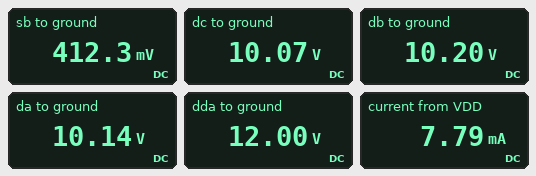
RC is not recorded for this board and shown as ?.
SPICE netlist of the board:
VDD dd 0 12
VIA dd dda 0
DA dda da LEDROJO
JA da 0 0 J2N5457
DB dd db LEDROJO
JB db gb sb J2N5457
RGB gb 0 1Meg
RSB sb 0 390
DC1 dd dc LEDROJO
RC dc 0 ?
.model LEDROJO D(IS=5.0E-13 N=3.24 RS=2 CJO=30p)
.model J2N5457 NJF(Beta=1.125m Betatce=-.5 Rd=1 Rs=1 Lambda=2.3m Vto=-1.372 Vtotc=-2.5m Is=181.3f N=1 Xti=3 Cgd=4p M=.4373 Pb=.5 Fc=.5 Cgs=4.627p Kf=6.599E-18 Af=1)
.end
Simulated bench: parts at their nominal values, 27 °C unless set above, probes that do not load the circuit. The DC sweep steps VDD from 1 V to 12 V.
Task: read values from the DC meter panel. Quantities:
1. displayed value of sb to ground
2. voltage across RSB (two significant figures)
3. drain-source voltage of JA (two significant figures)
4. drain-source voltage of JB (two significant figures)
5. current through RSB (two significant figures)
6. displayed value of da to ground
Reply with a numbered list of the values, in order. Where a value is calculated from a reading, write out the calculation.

1. 412.3 mV
2. 412.3 mV = 410 mV
3. 10.14 V = 10 V
4. 10.2 V - 412.3 mV = 9.8 V
5. (412.3 mV) / 390 Ω = 1.1 mA
6. 10.14 V
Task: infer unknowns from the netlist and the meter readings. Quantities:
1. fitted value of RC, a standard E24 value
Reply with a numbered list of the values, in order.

1. 2.2 kΩ
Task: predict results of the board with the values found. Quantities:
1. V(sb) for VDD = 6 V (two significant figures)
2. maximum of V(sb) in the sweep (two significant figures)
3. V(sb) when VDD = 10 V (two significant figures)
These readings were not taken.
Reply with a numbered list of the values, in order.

1. 410 mV
2. 410 mV
3. 410 mV
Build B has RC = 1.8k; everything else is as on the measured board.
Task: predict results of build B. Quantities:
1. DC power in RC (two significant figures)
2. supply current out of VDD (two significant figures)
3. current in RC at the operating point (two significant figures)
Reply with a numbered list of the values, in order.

1. 56 mW
2. 8.8 mA
3. 5.6 mA
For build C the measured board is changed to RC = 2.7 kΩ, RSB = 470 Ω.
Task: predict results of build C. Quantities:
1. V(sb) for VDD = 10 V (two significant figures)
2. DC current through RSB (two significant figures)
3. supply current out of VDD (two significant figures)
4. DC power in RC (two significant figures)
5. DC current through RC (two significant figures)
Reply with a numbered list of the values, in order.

1. 450 mV
2. 970 µA
3. 6.9 mA
4. 38 mW
5. 3.7 mA
